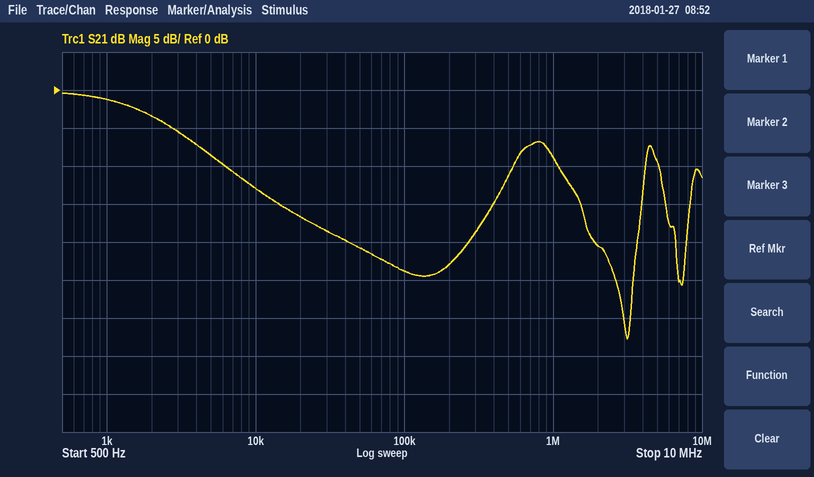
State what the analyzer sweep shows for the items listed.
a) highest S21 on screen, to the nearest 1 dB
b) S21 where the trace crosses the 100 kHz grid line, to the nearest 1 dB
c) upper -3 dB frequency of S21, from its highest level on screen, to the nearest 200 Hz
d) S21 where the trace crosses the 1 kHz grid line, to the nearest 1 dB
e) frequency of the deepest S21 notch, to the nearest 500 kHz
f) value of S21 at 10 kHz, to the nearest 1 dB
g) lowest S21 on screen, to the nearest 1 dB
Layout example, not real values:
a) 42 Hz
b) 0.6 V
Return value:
a) 0 dB
b) -24 dB
c) 2.0 kHz
d) -1 dB
e) 3.0 MHz
f) -13 dB
g) -33 dB
